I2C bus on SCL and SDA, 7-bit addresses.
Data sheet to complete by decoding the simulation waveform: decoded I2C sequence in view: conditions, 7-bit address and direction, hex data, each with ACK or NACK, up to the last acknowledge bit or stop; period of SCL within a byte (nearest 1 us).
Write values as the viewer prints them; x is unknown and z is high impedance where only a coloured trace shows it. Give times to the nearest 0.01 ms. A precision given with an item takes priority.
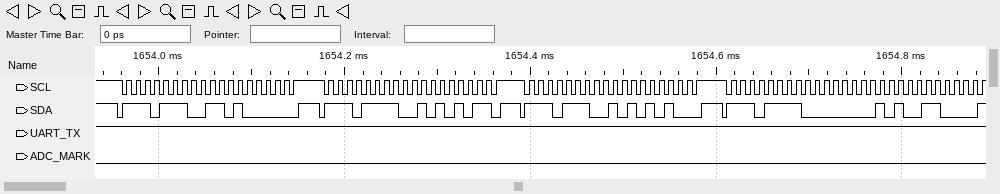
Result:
start, address 77 write ACK, D0 ACK, stop, start, address 77 read ACK, 55 NACK, stop, start, address 77 write ACK, AA ACK, stop, start, address 77 read ACK, 01 ACK, 98 ACK
10 us
